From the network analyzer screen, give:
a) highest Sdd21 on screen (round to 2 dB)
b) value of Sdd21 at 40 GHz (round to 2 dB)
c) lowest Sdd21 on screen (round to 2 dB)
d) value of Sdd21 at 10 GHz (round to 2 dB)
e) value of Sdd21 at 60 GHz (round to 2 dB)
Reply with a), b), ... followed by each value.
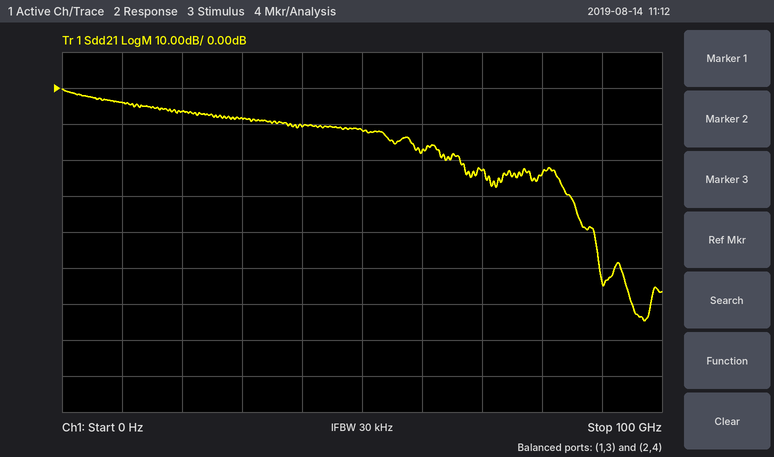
a) 0 dB
b) -10 dB
c) -64 dB
d) -4 dB
e) -18 dB
